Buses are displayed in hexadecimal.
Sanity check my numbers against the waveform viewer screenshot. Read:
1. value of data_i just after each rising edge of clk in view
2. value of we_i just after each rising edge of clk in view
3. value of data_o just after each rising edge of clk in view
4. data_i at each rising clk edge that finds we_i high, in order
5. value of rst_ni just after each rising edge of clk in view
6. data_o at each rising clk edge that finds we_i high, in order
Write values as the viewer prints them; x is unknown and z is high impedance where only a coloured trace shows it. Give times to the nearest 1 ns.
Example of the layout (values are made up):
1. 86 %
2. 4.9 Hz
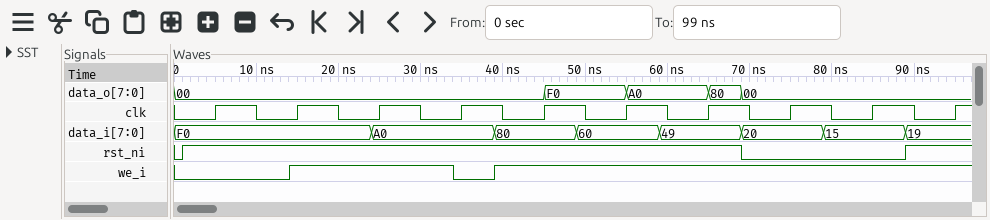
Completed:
1. F0, F0, A0, A0, 80, 60, 49, 20, 15, 19
2. 0 1 1 0 1 1 1 1 1 1
3. 00, 00, 00, 00, F0, A0, 80, 00, 00, 00
4. F0, A0, 80, 60, 49, 20, 15, 19
5. 1 1 1 1 1 1 1 0 0 1
6. 00, 00, 00, F0, A0, 00, 00, 00
